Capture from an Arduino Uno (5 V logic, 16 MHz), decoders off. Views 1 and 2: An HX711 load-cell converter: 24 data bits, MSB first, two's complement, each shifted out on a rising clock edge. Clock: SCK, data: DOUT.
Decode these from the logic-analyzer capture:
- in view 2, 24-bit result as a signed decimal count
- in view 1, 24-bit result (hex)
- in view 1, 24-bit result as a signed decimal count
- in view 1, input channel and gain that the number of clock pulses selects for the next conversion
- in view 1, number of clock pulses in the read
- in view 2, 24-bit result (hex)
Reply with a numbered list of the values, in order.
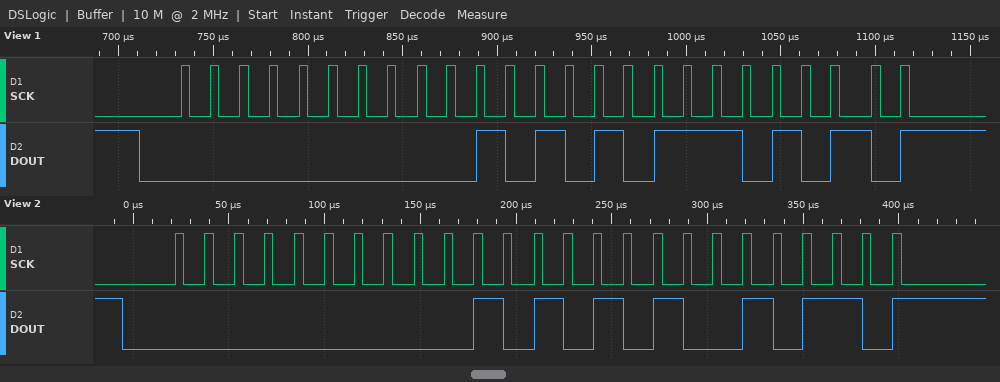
1. 10902
2. 0x002AEA
3. 10986
4. channel A, gain 128
5. 25
6. 0x002A96
